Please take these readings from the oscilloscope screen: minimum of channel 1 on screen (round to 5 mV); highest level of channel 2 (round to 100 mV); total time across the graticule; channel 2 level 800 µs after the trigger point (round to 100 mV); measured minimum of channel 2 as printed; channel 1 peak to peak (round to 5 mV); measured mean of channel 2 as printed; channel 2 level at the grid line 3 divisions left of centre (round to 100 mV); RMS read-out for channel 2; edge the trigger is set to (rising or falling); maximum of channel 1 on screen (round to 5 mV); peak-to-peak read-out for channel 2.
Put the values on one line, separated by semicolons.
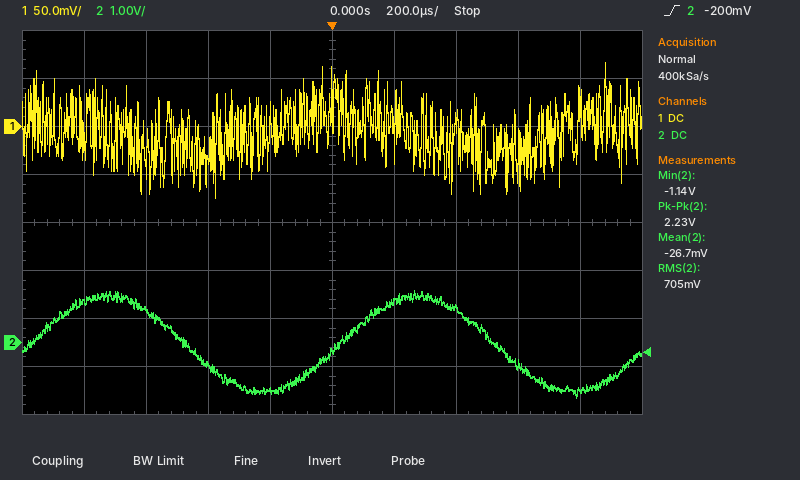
-75 mV; 1.1 V; 2 ms; -1.0 V; -1.14 V; 140 mV; -26.7 mV; 700 mV; 705 mV; rising; 65 mV; 2.23 V
